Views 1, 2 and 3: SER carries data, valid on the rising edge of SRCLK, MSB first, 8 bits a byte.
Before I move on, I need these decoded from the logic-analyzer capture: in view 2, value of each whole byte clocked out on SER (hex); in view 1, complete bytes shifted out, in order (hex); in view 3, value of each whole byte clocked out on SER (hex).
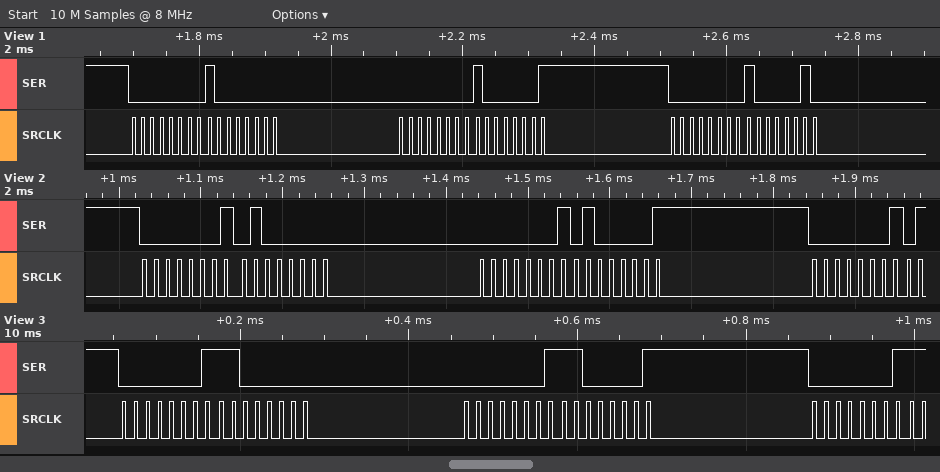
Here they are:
01 40 01 41 01
0x00 0x80 0x00 0x81 0x00 0x82
01 C0 01 C1 01
